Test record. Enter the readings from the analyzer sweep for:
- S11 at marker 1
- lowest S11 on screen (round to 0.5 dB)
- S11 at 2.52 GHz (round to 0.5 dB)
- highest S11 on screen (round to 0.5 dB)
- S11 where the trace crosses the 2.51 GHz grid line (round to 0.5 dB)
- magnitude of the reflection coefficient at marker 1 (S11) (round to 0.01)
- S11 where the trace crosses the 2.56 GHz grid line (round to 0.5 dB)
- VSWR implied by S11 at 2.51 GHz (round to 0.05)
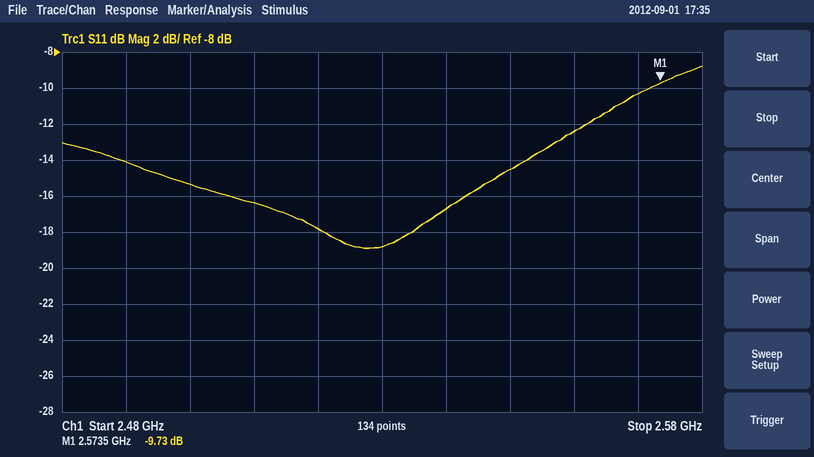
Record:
-9.73 dB
-19.0 dB
-18.0 dB
-9.0 dB
-16.5 dB
0.33
-12.5 dB
1.35
